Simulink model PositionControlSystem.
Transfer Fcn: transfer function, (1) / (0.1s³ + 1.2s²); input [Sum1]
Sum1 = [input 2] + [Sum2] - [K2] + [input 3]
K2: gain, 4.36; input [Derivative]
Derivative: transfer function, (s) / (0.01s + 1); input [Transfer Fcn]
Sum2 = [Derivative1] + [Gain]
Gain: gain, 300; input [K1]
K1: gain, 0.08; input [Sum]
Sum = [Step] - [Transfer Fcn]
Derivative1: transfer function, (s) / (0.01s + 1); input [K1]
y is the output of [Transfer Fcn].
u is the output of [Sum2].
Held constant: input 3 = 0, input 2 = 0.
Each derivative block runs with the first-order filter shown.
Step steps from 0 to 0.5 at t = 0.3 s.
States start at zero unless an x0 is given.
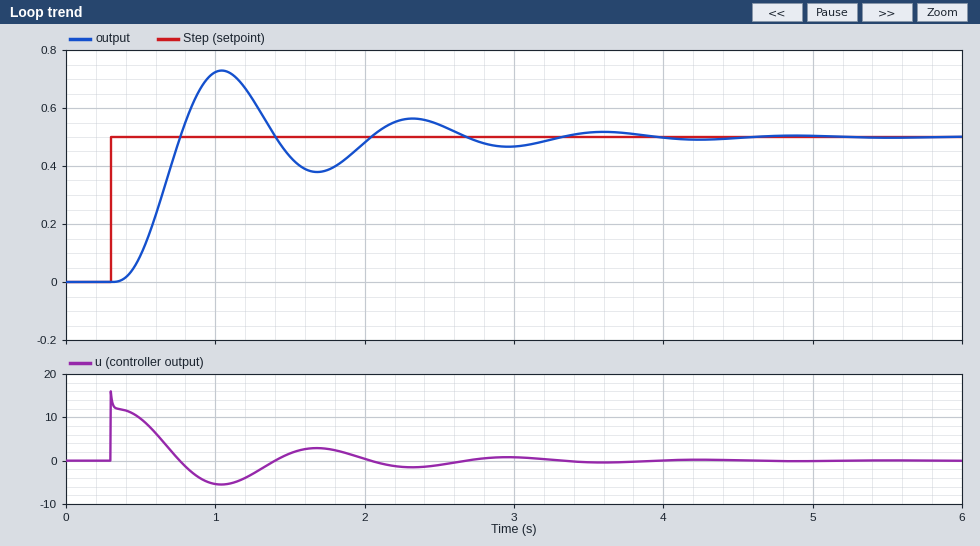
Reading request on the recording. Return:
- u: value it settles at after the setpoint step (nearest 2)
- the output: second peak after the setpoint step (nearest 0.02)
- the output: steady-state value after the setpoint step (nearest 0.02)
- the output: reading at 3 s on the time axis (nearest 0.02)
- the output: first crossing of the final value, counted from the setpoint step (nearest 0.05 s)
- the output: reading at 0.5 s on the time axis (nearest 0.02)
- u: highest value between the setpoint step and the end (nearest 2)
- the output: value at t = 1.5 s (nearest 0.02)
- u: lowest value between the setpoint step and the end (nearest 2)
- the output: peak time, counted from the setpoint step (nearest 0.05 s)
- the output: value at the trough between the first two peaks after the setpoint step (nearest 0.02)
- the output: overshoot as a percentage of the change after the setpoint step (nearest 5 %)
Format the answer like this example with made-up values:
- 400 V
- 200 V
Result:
- 0
- 0.56
- 0.50
- 0.46
- 0.45 s
- 0.10
- 16
- 0.44
- -6
- 0.75 s
- 0.38
- 45 %
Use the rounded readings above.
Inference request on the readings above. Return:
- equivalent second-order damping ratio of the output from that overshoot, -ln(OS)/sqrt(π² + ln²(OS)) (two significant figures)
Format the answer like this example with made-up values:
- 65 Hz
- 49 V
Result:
- 0.25
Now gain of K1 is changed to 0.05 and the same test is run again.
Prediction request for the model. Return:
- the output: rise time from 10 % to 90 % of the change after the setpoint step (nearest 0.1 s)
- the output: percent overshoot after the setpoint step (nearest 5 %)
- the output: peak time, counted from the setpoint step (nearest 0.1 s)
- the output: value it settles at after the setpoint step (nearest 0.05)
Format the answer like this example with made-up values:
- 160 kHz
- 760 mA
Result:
- 0.4 s
- 25 %
- 0.9 s
- 0.50
